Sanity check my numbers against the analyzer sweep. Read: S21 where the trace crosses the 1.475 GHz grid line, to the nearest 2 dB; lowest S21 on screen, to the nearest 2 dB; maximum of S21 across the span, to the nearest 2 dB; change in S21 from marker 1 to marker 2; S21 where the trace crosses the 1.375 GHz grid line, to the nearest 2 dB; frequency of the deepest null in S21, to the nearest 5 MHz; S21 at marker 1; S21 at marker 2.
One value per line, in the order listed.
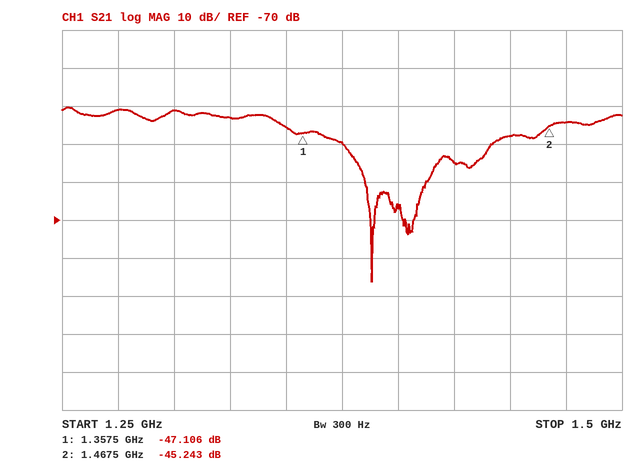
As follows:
-44 dB
-86 dB
-40 dB
1.863 dB
-50 dB
1.390 GHz
-47.106 dB
-45.243 dB
